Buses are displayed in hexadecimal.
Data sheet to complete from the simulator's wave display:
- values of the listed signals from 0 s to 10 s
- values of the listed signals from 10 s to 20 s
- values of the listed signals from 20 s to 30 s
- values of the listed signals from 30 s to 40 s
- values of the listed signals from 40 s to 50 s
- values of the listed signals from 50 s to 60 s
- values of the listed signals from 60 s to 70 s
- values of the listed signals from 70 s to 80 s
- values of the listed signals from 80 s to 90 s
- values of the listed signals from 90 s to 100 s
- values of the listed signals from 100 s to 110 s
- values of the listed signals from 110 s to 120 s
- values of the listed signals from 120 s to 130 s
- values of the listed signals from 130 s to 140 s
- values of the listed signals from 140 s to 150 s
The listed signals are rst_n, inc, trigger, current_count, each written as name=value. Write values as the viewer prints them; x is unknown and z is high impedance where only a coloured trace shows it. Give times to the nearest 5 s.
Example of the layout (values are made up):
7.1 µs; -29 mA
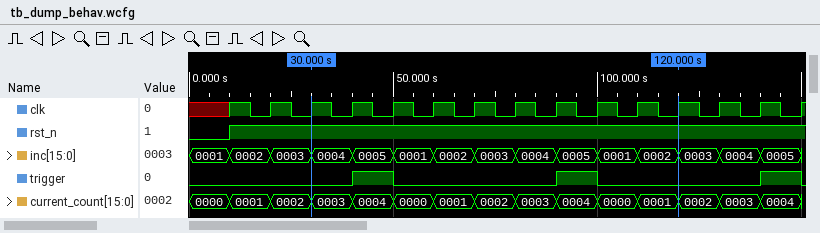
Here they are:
rst_n=0, inc=0001, trigger=0, current_count=0000; rst_n=1, inc=0002, trigger=0, current_count=0001; rst_n=1, inc=0003, trigger=0, current_count=0002; rst_n=1, inc=0004, trigger=0, current_count=0003; rst_n=1, inc=0005, trigger=1, current_count=0004; rst_n=1, inc=0001, trigger=0, current_count=0000; rst_n=1, inc=0002, trigger=0, current_count=0001; rst_n=1, inc=0003, trigger=0, current_count=0002; rst_n=1, inc=0004, trigger=0, current_count=0003; rst_n=1, inc=0005, trigger=1, current_count=0004; rst_n=1, inc=0001, trigger=0, current_count=0000; rst_n=1, inc=0002, trigger=0, current_count=0001; rst_n=1, inc=0003, trigger=0, current_count=0002; rst_n=1, inc=0004, trigger=0, current_count=0003; rst_n=1, inc=0005, trigger=1, current_count=0004
